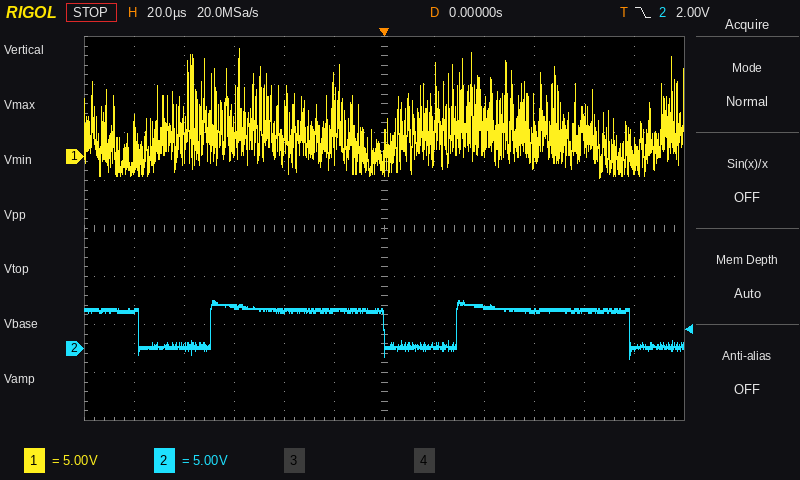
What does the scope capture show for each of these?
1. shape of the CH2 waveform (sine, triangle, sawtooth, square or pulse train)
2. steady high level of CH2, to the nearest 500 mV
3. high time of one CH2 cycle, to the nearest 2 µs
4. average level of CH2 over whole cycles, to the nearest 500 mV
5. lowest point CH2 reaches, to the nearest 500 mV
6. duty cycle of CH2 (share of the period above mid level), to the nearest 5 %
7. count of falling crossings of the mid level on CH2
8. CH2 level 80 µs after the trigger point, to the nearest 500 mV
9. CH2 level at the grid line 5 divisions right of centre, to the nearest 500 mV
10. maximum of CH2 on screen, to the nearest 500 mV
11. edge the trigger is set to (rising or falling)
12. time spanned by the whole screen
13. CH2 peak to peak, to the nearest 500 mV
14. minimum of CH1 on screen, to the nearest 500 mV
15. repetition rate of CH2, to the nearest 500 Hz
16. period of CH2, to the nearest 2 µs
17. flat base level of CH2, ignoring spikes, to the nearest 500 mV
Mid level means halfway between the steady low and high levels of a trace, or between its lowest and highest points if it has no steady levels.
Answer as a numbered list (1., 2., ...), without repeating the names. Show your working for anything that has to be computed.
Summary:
1. pulse train
2. 4.0 V
3. 70 µs
4. 0.0 V + 0.7 × (4.0 V − (0.0 V)) ≈ 2.80 V, so 3.0 V to the nearest 500 mV
5. -1.0 V
6. 70 µs / 98 µs ≈ 71.4 %, so 70 % to the nearest 5 %
7. 3
8. 4.0 V
9. 0.0 V
10. 5.0 V
11. falling
12. 240 µs
13. 5.0 V − (-1.0 V) = 6.0 V
14. -2.0 V
15. 1 / 98 µs ≈ 10.2 kHz, so 10.0 kHz to the nearest 500 Hz
16. 98 µs
17. 0.0 V
